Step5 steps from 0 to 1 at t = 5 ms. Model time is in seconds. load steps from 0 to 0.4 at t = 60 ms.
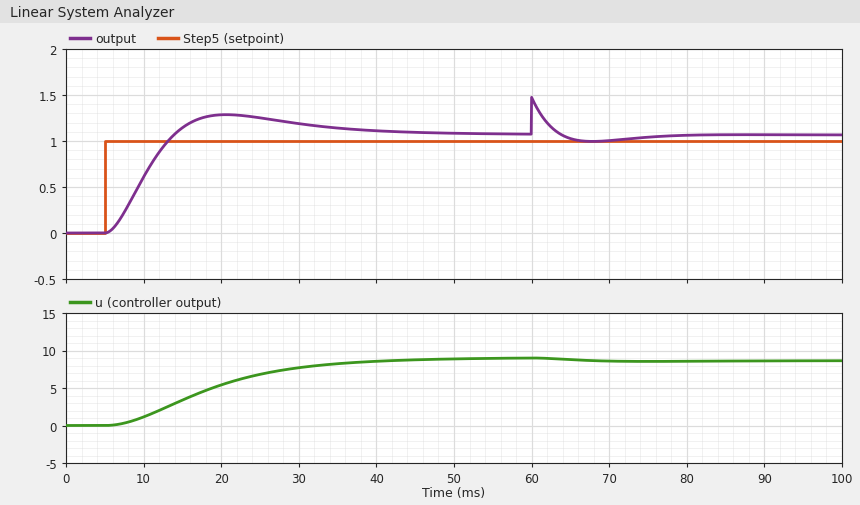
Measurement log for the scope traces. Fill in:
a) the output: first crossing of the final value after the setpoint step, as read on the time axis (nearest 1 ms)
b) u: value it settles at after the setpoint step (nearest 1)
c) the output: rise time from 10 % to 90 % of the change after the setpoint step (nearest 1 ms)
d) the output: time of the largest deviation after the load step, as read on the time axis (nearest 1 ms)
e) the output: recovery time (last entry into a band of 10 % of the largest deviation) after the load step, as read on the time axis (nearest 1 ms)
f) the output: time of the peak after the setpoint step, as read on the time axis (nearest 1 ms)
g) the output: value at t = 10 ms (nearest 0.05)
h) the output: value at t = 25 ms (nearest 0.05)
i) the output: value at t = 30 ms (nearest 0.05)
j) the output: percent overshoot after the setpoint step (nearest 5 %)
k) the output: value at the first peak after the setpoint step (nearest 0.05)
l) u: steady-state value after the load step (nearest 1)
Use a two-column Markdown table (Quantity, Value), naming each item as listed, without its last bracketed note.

| Quantity | Value |
|---|---|
| the output: first crossing of the final value after the setpoint step, as read on the time axis | 14 ms |
| u: value it settles at after the setpoint step | 9 |
| the output: rise time from 10 % to 90 % of the change after the setpoint step | 6 ms |
| the output: time of the largest deviation after the load step, as read on the time axis | 60 ms |
| the output: recovery time (last entry into a band of 10 % of the largest deviation) after the load step, as read on the time axis | 73 ms |
| the output: time of the peak after the setpoint step, as read on the time axis | 21 ms |
| the output: value at t = 10 ms | 0.60 |
| the output: value at t = 25 ms | 1.25 |
| the output: value at t = 30 ms | 1.20 |
| the output: percent overshoot after the setpoint step | 20 % |
| the output: value at the first peak after the setpoint step | 1.30 |
| u: steady-state value after the load step | 9 |
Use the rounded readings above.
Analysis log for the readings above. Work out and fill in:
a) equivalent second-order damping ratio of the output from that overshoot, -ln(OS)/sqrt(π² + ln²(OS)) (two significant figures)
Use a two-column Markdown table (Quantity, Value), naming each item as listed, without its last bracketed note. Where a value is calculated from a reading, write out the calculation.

| Quantity | Value |
|---|---|
| equivalent second-order damping ratio of the output from that overshoot, -ln(OS)/sqrt(π² + ln²(OS)) | ln(0.2) = -1.609; 1.609 / sqrt(9.870 + 2.590) = 0.46 |
